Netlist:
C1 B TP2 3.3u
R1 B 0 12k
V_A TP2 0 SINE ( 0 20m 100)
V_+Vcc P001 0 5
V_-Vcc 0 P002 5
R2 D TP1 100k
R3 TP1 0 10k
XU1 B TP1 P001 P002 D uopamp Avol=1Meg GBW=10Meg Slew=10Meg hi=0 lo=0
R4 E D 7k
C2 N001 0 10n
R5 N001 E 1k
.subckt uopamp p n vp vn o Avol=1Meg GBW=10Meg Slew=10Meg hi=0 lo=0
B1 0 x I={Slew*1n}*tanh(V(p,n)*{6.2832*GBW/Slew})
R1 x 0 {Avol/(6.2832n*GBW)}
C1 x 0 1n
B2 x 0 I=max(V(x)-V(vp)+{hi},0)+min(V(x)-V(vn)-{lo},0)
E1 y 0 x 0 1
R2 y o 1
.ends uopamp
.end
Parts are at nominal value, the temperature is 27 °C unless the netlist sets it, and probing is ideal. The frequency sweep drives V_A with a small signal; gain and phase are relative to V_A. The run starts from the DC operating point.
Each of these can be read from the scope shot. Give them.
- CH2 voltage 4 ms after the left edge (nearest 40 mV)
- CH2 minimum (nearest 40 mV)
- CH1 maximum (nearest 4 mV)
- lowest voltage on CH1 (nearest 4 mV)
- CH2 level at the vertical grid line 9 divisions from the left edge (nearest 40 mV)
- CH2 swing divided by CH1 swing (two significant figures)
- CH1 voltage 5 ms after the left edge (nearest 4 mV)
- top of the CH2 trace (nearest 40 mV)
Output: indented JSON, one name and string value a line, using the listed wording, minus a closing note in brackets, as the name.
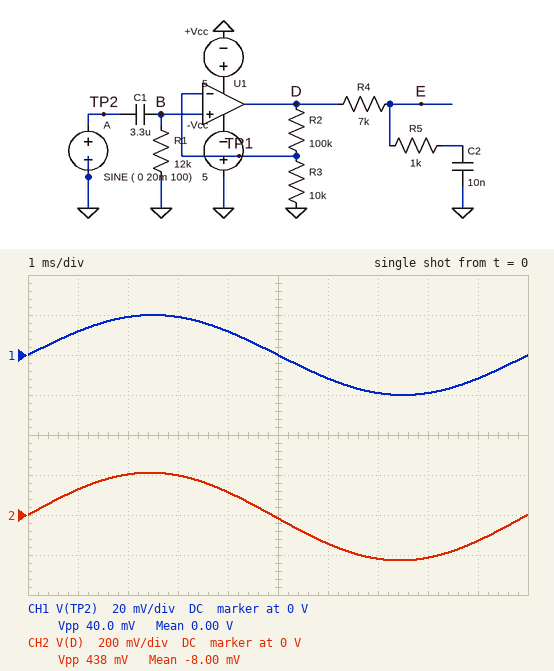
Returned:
{
  "CH2 voltage 4 ms after the left edge": "120 mV",
  "CH2 minimum": "-240 mV",
  "CH1 maximum": "20 mV",
  "lowest voltage on CH1": "-20 mV",
  "CH2 level at the vertical grid line 9 divisions from the left edge": "-120 mV",
  "CH2 swing divided by CH1 swing": "11",
  "CH1 voltage 5 ms after the left edge": "0 V",
  "top of the CH2 trace": "200 mV"
}
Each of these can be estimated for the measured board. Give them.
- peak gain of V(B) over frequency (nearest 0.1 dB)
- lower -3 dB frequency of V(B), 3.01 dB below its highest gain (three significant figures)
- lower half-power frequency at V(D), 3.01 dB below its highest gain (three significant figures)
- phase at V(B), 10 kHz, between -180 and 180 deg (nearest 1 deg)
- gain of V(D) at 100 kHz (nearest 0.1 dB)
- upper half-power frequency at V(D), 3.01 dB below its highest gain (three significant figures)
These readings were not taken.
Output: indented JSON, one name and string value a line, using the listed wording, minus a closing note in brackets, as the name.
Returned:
{
  "peak gain of V(B) over frequency": "0 dB",
  "lower -3 dB frequency of V(B), 3.01 dB below its highest gain": "4.02 Hz",
  "lower half-power frequency at V(D), 3.01 dB below its highest gain": "4.02 Hz",
  "phase at V(B), 10 kHz, between -180 and 180 deg": "0 deg",
  "gain of V(D) at 100 kHz": "20.8 dB",
  "upper half-power frequency at V(D), 3.01 dB below its highest gain": "909 kHz"
}
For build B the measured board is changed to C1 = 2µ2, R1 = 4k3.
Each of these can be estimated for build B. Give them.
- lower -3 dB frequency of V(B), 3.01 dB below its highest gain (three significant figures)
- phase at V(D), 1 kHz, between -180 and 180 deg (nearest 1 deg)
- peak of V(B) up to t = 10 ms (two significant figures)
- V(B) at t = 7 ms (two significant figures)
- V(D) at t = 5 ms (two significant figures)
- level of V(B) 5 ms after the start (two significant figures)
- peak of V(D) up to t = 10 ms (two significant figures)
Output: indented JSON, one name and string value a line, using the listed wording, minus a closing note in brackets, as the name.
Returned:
{
  "lower -3 dB frequency of V(B), 3.01 dB below its highest gain": "16.8 Hz",
  "phase at V(D), 1 kHz, between -180 and 180 deg": "1 deg",
  "peak of V(B) up to t = 10 ms": "17 mV",
  "V(B) at t = 7 ms": "-21 mV",
  "V(D) at t = 5 ms": "-57 mV",
  "level of V(B) 5 ms after the start": "-5.2 mV",
  "peak of V(D) up to t = 10 ms": "190 mV"
}
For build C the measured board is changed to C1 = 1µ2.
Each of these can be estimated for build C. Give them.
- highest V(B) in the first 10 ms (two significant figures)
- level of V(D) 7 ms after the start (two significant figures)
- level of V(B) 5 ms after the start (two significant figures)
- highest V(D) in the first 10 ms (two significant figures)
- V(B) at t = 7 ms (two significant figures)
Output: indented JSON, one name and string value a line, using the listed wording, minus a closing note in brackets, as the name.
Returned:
{
  "highest V(B) in the first 10 ms": "18 mV",
  "level of V(D) 7 ms after the start": "-230 mV",
  "level of V(B) 5 ms after the start": "-3.7 mV",
  "highest V(D) in the first 10 ms": "200 mV",
  "V(B) at t = 7 ms": "-21 mV"
}
